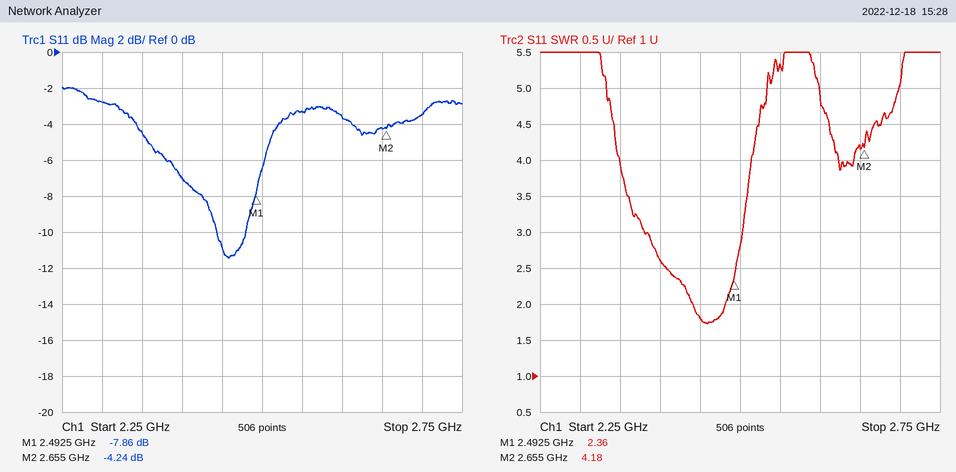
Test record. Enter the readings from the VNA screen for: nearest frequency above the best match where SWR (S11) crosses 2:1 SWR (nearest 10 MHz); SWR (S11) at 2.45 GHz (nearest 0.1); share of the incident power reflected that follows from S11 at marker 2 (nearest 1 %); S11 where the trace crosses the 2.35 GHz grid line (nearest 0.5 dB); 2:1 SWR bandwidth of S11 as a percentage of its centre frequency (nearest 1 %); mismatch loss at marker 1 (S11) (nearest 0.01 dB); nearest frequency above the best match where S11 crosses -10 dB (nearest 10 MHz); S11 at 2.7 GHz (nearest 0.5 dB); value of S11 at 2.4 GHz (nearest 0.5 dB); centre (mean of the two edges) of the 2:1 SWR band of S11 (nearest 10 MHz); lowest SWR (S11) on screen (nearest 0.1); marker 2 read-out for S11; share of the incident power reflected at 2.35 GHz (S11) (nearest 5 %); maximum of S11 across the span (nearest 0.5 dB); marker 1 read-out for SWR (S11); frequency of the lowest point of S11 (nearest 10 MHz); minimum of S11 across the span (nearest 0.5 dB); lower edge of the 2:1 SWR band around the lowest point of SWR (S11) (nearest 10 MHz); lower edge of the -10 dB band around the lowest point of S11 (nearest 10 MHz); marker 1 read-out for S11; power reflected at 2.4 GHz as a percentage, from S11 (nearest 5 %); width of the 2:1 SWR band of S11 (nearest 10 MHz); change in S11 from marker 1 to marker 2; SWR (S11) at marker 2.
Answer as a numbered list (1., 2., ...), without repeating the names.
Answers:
1. 2.48 GHz
2. 1.8
3. 38 %
4. -4.5 dB
5. 2 %
6. 0.78 dB
7. 2.48 GHz
8. -3.5 dB
9. -7.0 dB
10. 2.46 GHz
11. 1.7
12. -4.24 dB
13. 35 %
14. -2.0 dB
15. 2.36
16. 2.46 GHz
17. -11.5 dB
18. 2.44 GHz
19. 2.44 GHz
20. -7.86 dB
21. 20 %
22. 40 MHz
23. 3.62 dB
24. 4.18
